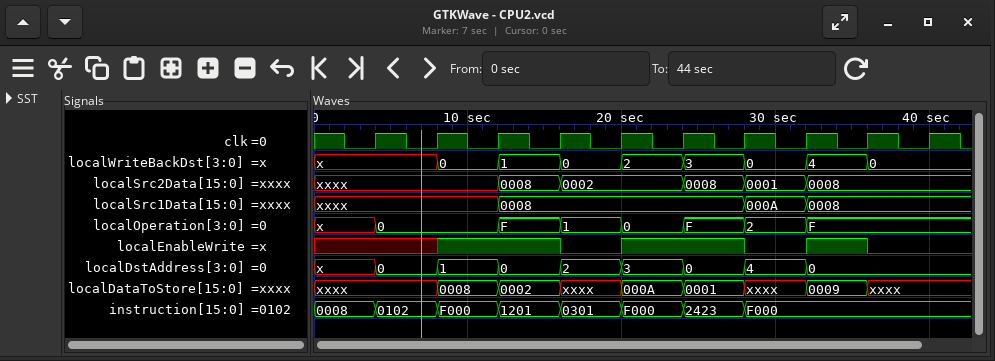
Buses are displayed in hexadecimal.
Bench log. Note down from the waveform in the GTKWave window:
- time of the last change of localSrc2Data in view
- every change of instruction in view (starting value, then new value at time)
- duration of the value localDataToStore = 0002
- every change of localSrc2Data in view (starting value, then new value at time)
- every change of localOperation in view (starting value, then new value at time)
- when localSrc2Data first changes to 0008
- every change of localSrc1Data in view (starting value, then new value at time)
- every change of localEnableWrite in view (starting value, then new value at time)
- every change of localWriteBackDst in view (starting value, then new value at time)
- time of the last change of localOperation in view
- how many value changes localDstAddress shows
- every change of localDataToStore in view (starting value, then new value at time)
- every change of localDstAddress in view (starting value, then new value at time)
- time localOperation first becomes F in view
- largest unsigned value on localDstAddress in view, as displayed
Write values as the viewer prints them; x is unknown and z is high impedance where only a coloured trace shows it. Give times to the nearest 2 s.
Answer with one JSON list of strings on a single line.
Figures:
["32 s", "0008, 0102 at 4 s, F000 at 8 s, 1201 at 12 s, 0301 at 16 s, F000 at 20 s, 2423 at 24 s, F000 at 28 s", "4 s", "xxxx, 0008 at 12 s, 0002 at 16 s, 0008 at 24 s, 0001 at 28 s, 0008 at 32 s", "x, 0 at 4 s, F at 12 s, 1 at 16 s, 0 at 20 s, F at 24 s, 2 at 28 s, F at 32 s", "12 s", "xxxx, 0008 at 12 s, 000A at 28 s, 0008 at 32 s", "x, 1 at 8 s, 0 at 16 s, 1 at 20 s, 0 at 28 s, 1 at 32 s, 0 at 36 s", "x, 0 at 8 s, 1 at 12 s, 0 at 16 s, 2 at 20 s, 3 at 24 s, 0 at 28 s, 4 at 32 s, 0 at 36 s", "32 s", "8", "xxxx, 0008 at 8 s, 0002 at 12 s, xxxx at 16 s, 000A at 20 s, 0001 at 24 s, xxxx at 28 s, 0009 at 32 s, xxxx at 36 s", "x, 0 at 4 s, 1 at 8 s, 0 at 12 s, 2 at 16 s, 3 at 20 s, 0 at 24 s, 4 at 28 s, 0 at 32 s", "12 s", "4"]
